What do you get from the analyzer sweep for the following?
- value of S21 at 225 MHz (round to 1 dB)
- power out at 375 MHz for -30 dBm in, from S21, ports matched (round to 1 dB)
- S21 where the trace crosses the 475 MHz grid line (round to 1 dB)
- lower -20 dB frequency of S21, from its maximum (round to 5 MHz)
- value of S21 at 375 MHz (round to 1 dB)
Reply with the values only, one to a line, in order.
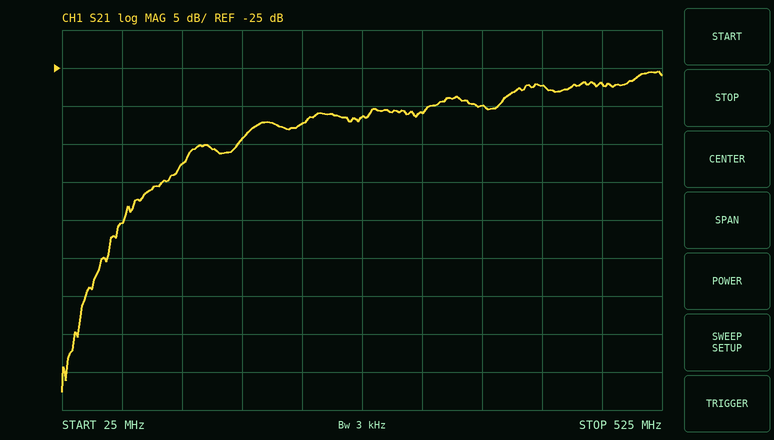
-32 dB
-60 dBm
-27 dB
75 MHz
-30 dB
